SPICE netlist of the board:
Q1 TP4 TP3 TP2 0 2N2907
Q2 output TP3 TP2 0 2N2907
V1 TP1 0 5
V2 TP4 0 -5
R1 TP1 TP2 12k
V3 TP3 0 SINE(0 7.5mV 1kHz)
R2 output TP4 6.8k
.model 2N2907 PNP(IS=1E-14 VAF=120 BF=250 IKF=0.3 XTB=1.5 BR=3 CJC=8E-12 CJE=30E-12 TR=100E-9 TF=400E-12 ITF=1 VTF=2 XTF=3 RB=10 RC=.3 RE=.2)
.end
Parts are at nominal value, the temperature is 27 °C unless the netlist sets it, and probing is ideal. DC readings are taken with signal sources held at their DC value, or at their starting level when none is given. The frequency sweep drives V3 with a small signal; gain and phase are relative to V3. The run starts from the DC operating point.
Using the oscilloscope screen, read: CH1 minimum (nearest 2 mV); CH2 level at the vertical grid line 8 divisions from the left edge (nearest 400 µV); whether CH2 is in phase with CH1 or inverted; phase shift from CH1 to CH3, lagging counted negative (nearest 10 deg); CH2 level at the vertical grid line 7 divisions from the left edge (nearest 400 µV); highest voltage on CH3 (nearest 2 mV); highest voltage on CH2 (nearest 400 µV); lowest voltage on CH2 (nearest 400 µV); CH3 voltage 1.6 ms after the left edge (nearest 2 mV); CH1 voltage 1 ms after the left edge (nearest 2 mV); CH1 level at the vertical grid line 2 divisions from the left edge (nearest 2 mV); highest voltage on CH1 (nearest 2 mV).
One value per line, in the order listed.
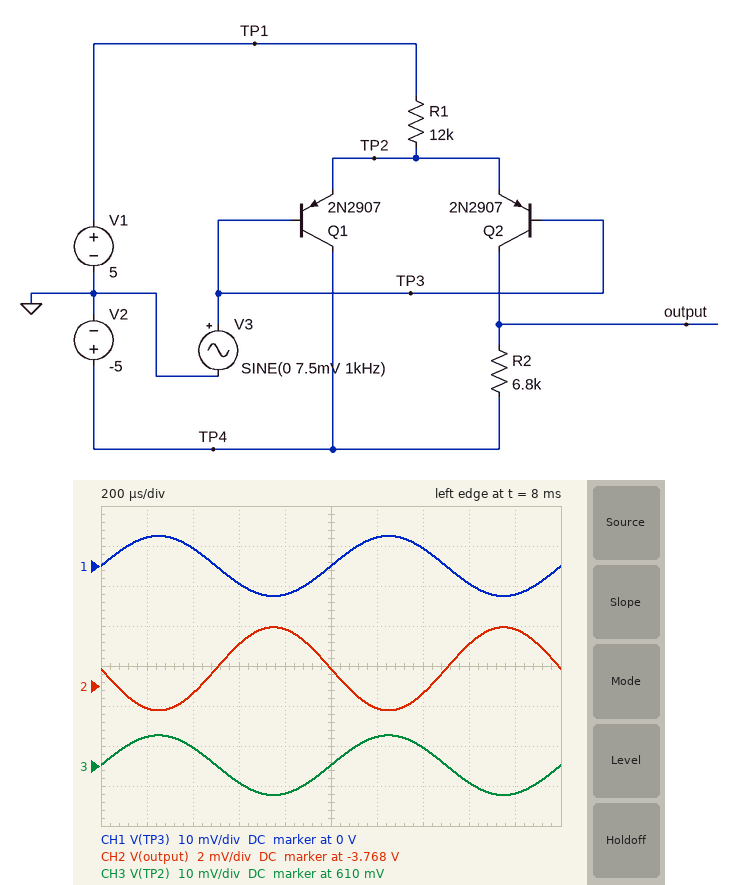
-8 mV
-3.7660 V
inverted
0 deg
-3.7684 V
618 mV
-3.7652 V
-3.7692 V
606 mV
0 V
4 mV
8 mV
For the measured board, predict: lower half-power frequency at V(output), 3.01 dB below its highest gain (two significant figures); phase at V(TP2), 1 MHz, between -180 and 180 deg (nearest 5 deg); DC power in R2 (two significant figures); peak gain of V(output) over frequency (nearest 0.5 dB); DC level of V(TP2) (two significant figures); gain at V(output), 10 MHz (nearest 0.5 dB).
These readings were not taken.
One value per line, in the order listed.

4.7 MHz
0 deg
220 µW
0 dB
610 mV
-1.0 dB
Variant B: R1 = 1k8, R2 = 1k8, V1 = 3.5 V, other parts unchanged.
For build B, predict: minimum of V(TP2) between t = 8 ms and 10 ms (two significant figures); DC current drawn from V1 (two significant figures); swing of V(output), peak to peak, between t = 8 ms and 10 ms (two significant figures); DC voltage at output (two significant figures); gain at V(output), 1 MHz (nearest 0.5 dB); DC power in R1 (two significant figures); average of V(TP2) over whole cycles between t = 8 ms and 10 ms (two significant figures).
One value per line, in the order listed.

640 mV
1.6 mA
7.3 mV
-3.6 V
-6.0 dB
4.5 mW
650 mV
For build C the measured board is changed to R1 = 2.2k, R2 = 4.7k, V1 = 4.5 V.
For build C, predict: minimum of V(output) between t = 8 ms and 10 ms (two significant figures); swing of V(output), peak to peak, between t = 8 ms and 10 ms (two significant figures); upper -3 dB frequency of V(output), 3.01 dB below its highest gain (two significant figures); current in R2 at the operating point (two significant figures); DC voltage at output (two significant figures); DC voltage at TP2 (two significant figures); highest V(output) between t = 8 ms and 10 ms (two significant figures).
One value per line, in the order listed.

-980 mV
15 mV
7.6 GHz
860 µA
-970 mV
650 mV
-960 mV
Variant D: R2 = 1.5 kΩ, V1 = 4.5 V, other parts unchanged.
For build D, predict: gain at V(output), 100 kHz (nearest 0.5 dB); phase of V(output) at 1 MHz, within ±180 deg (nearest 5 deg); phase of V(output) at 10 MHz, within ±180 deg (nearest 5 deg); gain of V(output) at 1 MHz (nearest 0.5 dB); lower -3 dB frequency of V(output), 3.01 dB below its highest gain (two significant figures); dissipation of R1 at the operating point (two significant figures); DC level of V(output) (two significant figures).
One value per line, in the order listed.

-24.0 dB
145 deg
75 deg
-22.5 dB
26 MHz
1.3 mW
-4.8 V
